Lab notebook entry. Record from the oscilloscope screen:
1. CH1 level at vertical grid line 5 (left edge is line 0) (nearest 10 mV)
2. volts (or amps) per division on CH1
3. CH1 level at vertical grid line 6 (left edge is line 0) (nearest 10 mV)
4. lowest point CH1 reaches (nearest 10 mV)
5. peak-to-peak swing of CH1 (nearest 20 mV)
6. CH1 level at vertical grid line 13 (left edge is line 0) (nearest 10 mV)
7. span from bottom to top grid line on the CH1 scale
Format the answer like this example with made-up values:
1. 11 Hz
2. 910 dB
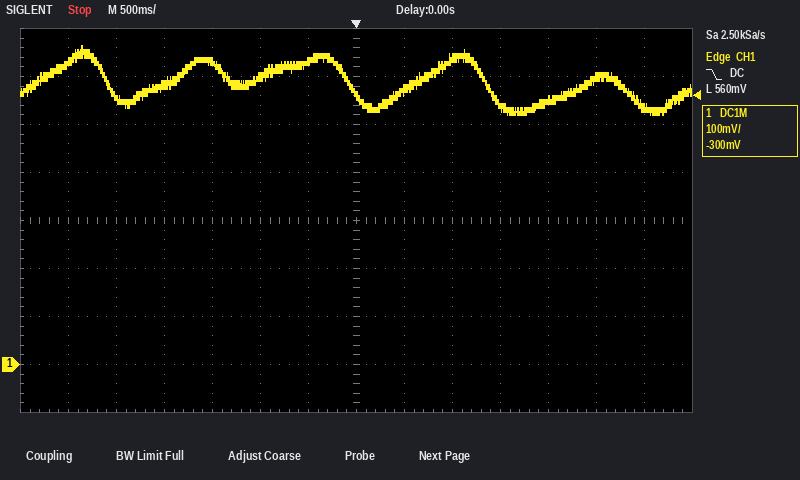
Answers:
1. 600 mV
2. 100 mV
3. 630 mV
4. 520 mV
5. 140 mV
6. 540 mV
7. 800 mV
